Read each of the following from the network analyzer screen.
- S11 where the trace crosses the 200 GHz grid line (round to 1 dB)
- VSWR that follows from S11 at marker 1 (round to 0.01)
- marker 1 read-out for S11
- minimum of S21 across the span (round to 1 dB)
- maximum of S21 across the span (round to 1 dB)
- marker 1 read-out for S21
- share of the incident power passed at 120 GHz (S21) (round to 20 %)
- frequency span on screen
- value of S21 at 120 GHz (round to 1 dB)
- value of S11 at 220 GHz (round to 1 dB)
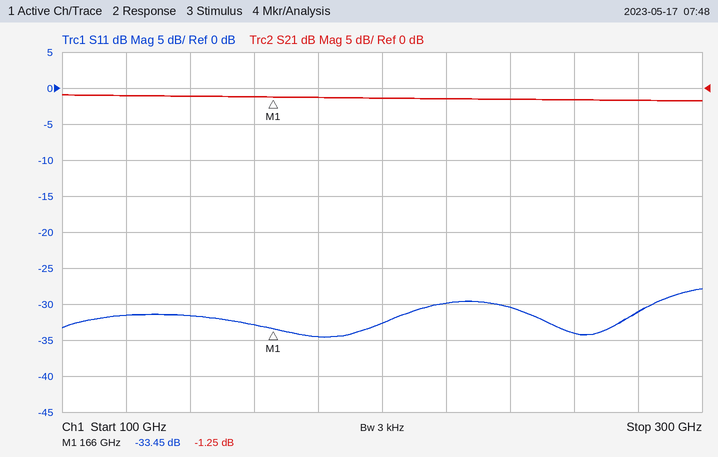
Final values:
-33 dB
1.04
-33.45 dB
-2 dB
-1 dB
-1.25 dB
80 %
200 GHz
-1 dB
-30 dB
